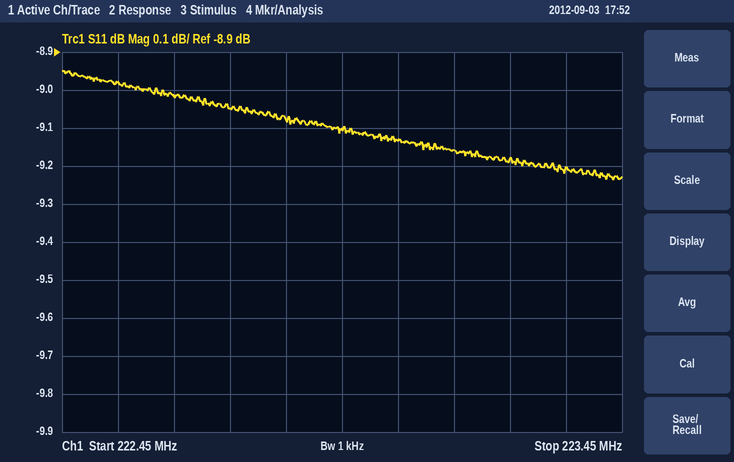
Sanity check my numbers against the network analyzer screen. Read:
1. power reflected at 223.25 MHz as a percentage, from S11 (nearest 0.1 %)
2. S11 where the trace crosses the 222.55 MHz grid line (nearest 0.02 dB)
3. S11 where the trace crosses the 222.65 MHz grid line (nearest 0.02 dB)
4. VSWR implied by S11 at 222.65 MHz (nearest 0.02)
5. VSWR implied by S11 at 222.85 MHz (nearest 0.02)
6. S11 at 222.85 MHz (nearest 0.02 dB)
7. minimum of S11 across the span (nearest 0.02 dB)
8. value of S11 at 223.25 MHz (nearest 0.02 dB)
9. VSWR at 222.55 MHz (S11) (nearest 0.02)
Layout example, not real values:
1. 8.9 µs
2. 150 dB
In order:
1. 12.1 %
2. -8.98 dB
3. -9.02 dB
4. 2.10
5. 2.08
6. -9.08 dB
7. -9.24 dB
8. -9.18 dB
9. 2.10
